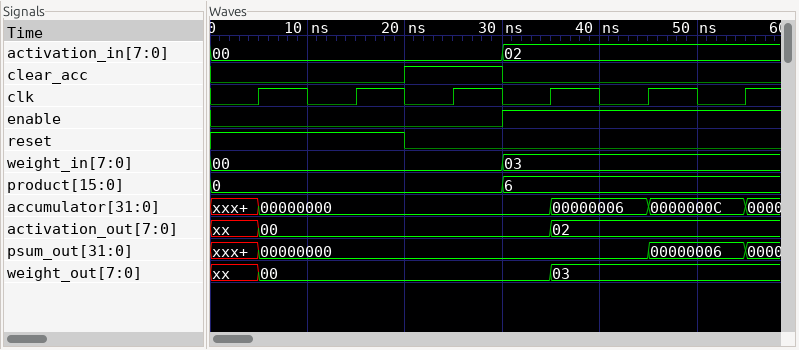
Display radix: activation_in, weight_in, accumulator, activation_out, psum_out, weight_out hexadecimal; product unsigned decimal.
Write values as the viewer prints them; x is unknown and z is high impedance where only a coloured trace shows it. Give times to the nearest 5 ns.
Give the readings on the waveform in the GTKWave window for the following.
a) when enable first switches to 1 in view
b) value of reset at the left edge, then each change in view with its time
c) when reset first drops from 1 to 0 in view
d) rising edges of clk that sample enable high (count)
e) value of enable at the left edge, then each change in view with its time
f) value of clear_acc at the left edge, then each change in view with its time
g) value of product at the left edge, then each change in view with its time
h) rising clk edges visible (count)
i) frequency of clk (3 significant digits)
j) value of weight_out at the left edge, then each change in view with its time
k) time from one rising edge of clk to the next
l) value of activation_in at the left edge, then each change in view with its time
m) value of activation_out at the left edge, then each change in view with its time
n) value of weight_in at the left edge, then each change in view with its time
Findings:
30 ns
1, 0 at 20 ns
20 ns
3
0, 1 at 30 ns
0, 1 at 20 ns, 0 at 30 ns
0, 6 at 30 ns
6
100 MHz
xx, 00 at 5 ns, 03 at 35 ns
10 ns
00, 02 at 30 ns
xx, 00 at 5 ns, 02 at 35 ns
00, 03 at 30 ns
